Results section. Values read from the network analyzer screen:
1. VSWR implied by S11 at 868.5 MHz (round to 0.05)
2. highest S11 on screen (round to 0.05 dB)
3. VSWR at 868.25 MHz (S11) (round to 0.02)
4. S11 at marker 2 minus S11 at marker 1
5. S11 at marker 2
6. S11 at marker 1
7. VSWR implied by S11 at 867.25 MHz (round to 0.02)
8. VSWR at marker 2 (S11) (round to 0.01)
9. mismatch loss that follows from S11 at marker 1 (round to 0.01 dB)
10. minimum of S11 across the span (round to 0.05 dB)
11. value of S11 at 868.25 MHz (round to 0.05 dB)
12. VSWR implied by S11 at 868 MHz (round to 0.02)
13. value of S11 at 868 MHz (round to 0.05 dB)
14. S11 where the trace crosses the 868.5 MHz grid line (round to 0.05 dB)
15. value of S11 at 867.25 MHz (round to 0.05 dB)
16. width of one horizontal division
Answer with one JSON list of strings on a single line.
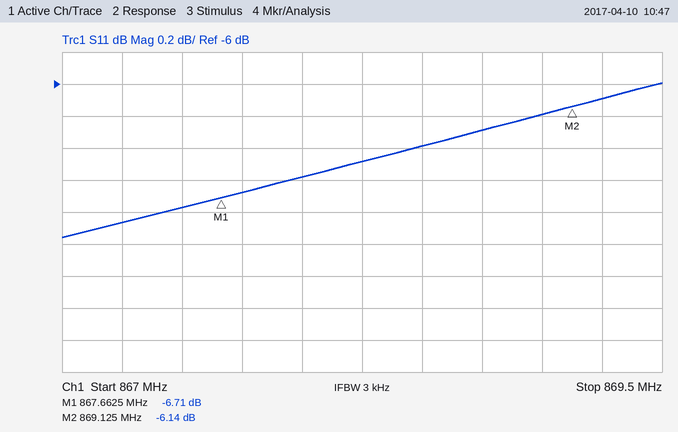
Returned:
["2.85", "-6.00 dB", "2.80", "0.57 dB", "-6.14 dB", "-6.71 dB", "2.66", "2.95", "1.04 dB", "-6.95 dB", "-6.50 dB", "2.76", "-6.60 dB", "-6.40 dB", "-6.85 dB", "250 kHz"]
